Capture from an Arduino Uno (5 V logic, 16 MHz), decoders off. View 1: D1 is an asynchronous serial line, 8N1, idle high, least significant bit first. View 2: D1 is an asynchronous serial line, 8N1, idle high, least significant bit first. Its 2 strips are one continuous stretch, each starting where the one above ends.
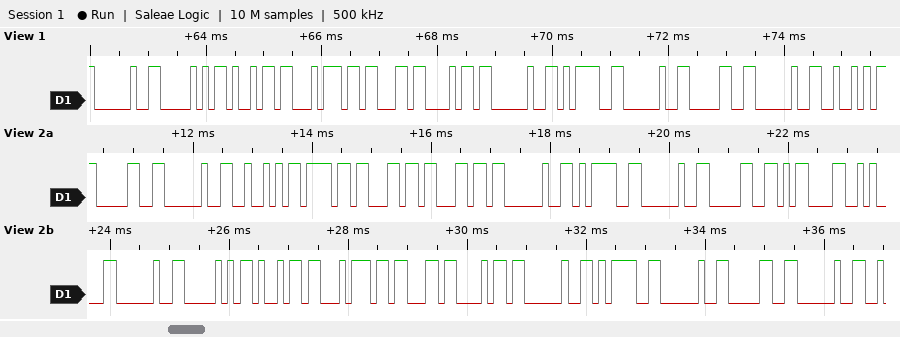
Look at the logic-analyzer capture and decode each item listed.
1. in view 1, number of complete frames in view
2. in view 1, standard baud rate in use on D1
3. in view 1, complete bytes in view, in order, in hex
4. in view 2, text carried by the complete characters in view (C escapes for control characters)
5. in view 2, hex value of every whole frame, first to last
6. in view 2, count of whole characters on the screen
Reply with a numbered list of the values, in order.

1. 12
2. 9600 baud
3. 0x20 0x50 0x69 0x74 0x63 0x68 0x20 0x3D 0x20 0x30 0x20 0x52
4. "0 Roll = 0\r\n Pitch = 0 "
5. 30 20 52 6F 6C 6C 20 3D 20 30 0D 0A 20 50 69 74 63 68 20 3D 20 30 20
6. 23
